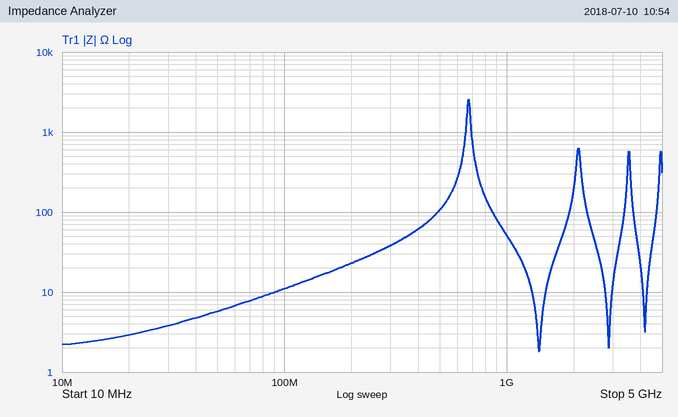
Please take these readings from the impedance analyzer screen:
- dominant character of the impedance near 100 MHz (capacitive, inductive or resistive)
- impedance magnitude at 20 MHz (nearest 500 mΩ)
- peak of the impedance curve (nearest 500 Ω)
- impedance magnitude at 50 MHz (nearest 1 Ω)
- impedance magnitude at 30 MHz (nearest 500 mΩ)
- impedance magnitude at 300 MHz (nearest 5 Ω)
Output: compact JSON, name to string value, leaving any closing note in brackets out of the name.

{"dominant character of the impedance near 100 MHz": "inductive", "impedance magnitude at 20 MHz": "3.0 Ω", "peak of the impedance curve": "2.5 kΩ", "impedance magnitude at 50 MHz": "6 Ω", "impedance magnitude at 30 MHz": "4.0 Ω", "impedance magnitude at 300 MHz": "40 Ω"}
